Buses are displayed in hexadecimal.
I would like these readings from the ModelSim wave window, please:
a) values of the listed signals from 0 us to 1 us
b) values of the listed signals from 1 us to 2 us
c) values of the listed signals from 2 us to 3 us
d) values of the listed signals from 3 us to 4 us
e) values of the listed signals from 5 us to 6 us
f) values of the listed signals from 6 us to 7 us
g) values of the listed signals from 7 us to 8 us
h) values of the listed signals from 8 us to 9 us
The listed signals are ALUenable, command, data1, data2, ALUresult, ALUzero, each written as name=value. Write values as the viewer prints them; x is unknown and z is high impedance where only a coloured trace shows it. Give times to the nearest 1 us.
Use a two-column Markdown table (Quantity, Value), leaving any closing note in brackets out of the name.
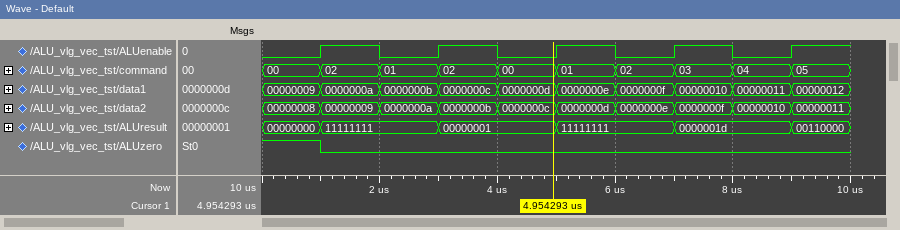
| Quantity | Value |
|---|---|
| values of the listed signals from 0 us to 1 us | ALUenable=0, command=00, data1=00000009, data2=00000008, ALUresult=00000000, ALUzero=1 |
| values of the listed signals from 1 us to 2 us | ALUenable=1, command=02, data1=0000000a, data2=00000009, ALUresult=11111111, ALUzero=0 |
| values of the listed signals from 2 us to 3 us | ALUenable=0, command=01, data1=0000000b, data2=0000000a, ALUresult=11111111, ALUzero=0 |
| values of the listed signals from 3 us to 4 us | ALUenable=1, command=02, data1=0000000c, data2=0000000b, ALUresult=00000001, ALUzero=0 |
| values of the listed signals from 5 us to 6 us | ALUenable=1, command=01, data1=0000000e, data2=0000000d, ALUresult=11111111, ALUzero=0 |
| values of the listed signals from 6 us to 7 us | ALUenable=0, command=02, data1=0000000f, data2=0000000e, ALUresult=11111111, ALUzero=0 |
| values of the listed signals from 7 us to 8 us | ALUenable=1, command=03, data1=00000010, data2=0000000f, ALUresult=0000001d, ALUzero=0 |
| values of the listed signals from 8 us to 9 us | ALUenable=0, command=04, data1=00000011, data2=00000010, ALUresult=0000001d, ALUzero=0 |
